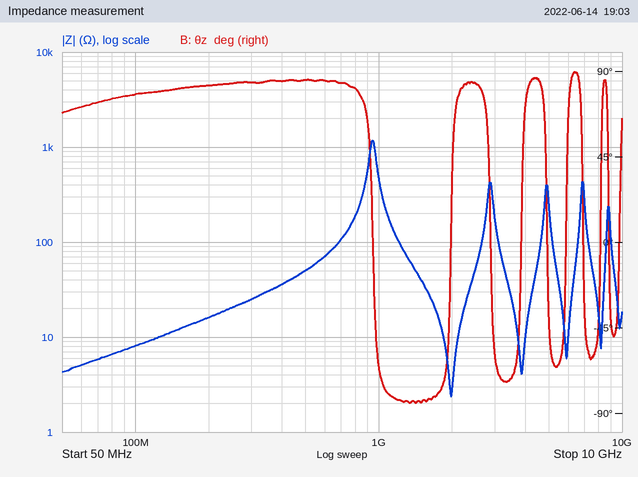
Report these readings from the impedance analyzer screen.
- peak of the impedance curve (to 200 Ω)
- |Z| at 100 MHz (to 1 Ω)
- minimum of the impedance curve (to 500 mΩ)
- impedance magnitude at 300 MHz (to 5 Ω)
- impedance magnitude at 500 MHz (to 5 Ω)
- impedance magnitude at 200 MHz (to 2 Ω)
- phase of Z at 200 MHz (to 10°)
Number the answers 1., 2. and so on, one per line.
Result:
1. 1.2 kΩ
2. 8 Ω
3. 2.5 Ω
4. 25 Ω
5. 50 Ω
6. 16 Ω
7. 80°
